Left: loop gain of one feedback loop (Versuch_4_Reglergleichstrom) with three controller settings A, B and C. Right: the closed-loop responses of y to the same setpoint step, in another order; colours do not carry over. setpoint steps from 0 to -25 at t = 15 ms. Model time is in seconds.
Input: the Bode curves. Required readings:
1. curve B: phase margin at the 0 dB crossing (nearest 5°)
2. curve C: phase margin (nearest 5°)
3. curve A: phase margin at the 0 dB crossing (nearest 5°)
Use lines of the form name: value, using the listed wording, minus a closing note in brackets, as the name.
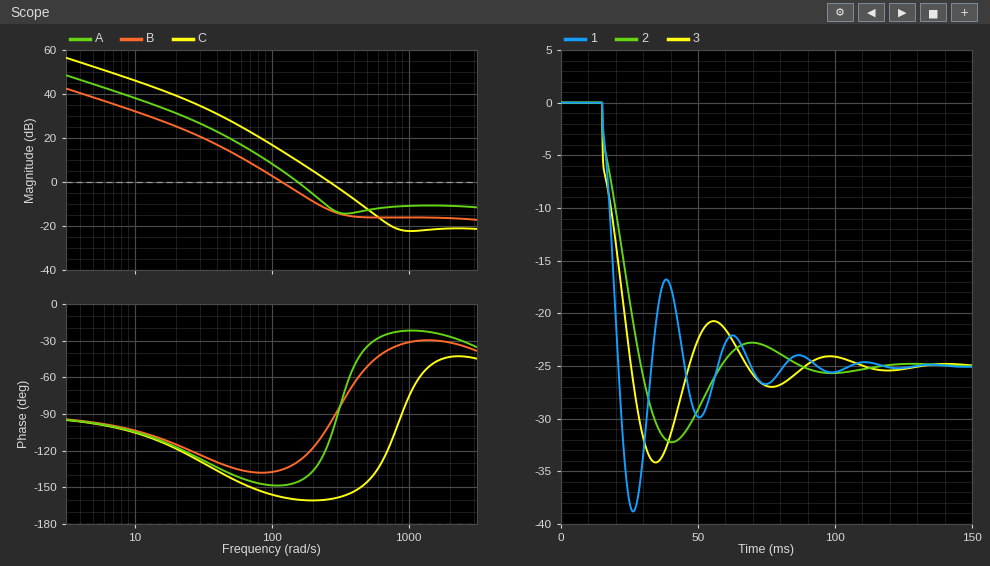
curve B: phase margin at the 0 dB crossing: 45°
curve C: phase margin: 20°
curve A: phase margin at the 0 dB crossing: 35°
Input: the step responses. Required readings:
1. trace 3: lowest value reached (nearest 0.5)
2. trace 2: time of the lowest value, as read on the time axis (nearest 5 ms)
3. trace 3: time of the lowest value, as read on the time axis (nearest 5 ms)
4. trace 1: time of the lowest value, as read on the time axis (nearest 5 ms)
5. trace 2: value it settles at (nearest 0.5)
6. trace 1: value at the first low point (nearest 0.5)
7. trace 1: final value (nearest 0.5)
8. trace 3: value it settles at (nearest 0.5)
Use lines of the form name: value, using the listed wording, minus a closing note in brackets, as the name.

trace 3: lowest value reached: -34.0
trace 2: time of the lowest value, as read on the time axis: 40 ms
trace 3: time of the lowest value, as read on the time axis: 35 ms
trace 1: time of the lowest value, as read on the time axis: 25 ms
trace 2: value it settles at: -25.0
trace 1: value at the first low point: -39.0
trace 1: final value: -25.0
trace 3: value it settles at: -25.0
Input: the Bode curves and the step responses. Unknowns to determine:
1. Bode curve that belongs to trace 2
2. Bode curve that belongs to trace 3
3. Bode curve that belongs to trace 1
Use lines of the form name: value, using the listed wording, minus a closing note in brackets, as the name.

Bode curve that belongs to trace 2: B
Bode curve that belongs to trace 3: A
Bode curve that belongs to trace 1: C
